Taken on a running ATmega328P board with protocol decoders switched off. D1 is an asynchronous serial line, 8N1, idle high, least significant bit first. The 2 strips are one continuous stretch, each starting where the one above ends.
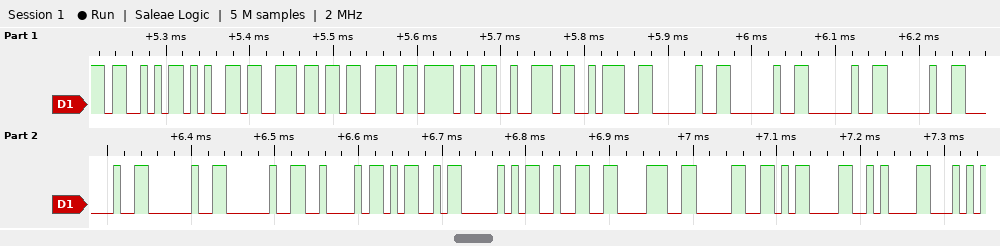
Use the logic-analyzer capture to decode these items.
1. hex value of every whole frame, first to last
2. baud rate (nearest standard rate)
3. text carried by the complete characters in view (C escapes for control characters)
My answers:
53 65 6E 73 6F 72 3A 20 20 20 20 20 20 20 42 4D 50 32 38 30 0D 0A
115200 baud
"Sensor:       BMP280\r\n"
